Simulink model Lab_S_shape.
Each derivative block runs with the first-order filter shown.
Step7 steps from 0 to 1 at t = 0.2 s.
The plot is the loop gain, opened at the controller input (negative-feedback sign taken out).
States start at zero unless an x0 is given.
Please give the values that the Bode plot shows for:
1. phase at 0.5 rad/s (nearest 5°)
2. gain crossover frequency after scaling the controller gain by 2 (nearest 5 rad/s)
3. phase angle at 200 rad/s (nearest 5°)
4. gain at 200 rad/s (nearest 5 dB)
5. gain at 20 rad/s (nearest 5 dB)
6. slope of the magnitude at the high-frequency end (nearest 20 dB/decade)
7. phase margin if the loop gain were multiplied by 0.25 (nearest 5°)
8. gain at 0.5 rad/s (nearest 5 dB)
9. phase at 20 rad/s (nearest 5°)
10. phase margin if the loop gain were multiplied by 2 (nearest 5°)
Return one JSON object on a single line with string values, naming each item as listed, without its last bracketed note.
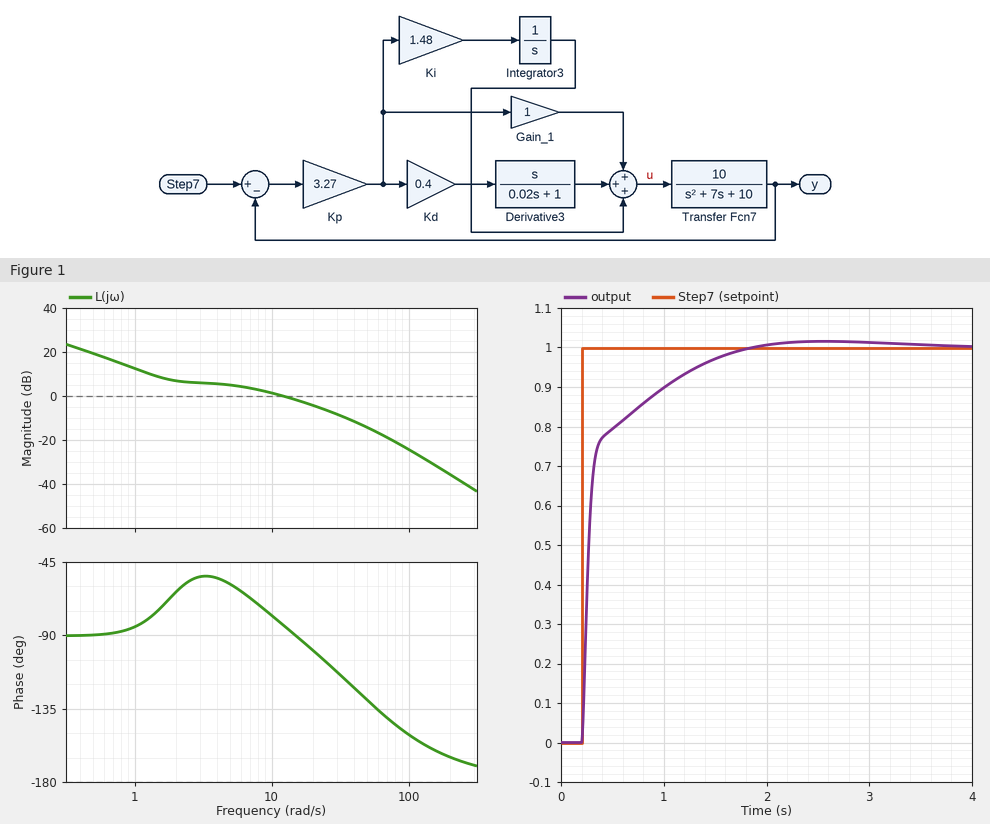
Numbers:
{"phase at 0.5 rad/s": "-90°", "gain crossover frequency after scaling the controller gain by 2": "25 rad/s", "phase angle at 200 rad/s": "-165°", "gain at 200 rad/s": "-35 dB", "gain at 20 rad/s": "-5 dB", "slope of the magnitude at the high-frequency end": "-40 dB/decade", "phase margin if the loop gain were multiplied by 0.25": "95°", "gain at 0.5 rad/s": "20 dB", "phase at 20 rad/s": "-100°", "phase margin if the loop gain were multiplied by 2": "75°"}
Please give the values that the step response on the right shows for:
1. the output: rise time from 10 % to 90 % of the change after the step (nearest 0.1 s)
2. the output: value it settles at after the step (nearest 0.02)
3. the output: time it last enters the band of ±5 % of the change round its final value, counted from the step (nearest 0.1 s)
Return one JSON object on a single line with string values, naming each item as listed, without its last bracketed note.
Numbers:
{"the output: rise time from 10 % to 90 % of the change after the step": "0.8 s", "the output: value it settles at after the step": "1.00", "the output: time it last enters the band of ±5 % of the change round its final value, counted from the step": "1.1 s"}
